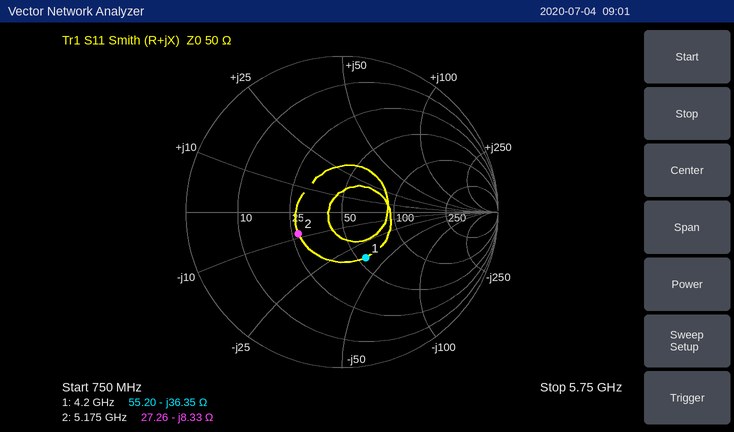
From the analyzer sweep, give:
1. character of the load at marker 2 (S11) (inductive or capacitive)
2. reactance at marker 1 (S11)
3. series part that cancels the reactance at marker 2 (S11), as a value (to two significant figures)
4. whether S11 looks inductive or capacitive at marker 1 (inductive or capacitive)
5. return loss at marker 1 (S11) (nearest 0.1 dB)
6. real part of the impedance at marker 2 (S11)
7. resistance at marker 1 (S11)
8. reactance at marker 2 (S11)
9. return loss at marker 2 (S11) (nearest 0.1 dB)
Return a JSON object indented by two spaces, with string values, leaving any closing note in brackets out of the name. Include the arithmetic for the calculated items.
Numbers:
{
  "character of the load at marker 2 (S11)": "capacitive",
  "reactance at marker 1": "-36.35 Ω",
  "series part that cancels the reactance at marker 2 (S11), as a value": "L = 8.33 Ω/(2π × 5.175 GHz) ≈ 256 pH, so 260 pH to two significant figures",
  "whether S11 looks inductive or capacitive at marker 1": "capacitive",
  "return loss at marker 1 (S11)": "9.6 dB",
  "real part of the impedance at marker 2": "27.26 Ω",
  "resistance at marker 1": "55.20 Ω",
  "reactance at marker 2": "-8.33 Ω",
  "return loss at marker 2 (S11)": "10.1 dB"
}
